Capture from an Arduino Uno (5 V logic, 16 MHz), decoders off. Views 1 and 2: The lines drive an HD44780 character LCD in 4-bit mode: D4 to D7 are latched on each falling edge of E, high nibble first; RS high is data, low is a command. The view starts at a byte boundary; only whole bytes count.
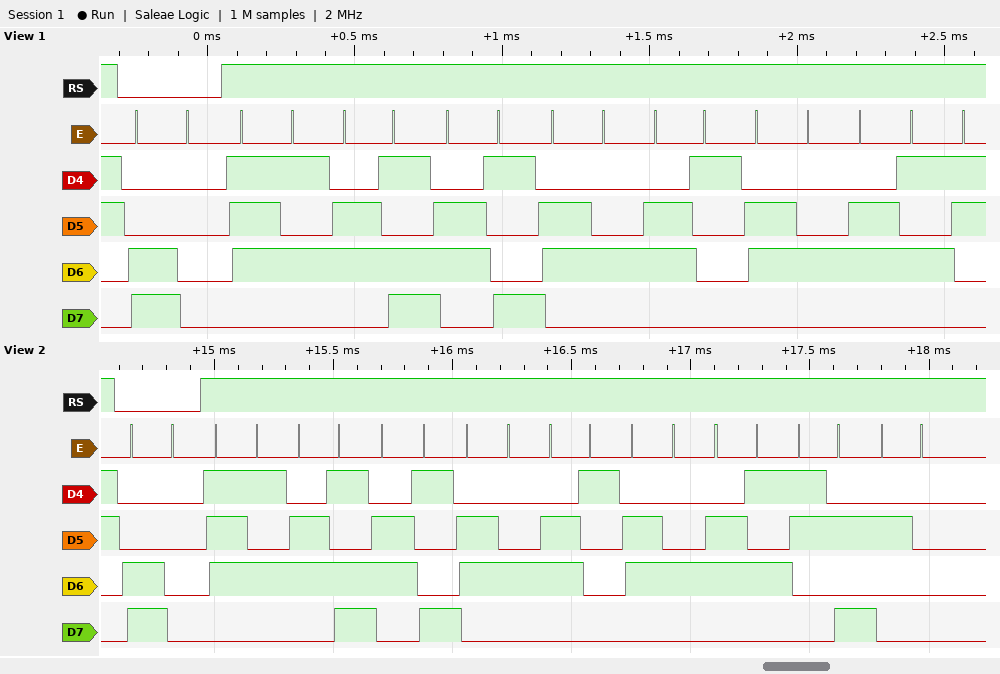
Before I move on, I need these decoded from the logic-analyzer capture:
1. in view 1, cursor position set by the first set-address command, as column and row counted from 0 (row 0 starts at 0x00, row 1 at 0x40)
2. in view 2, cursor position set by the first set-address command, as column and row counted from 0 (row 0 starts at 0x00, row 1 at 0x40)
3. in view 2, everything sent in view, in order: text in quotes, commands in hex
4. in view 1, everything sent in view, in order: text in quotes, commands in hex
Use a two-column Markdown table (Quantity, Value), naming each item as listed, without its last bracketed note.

| Quantity | Value |
|---|---|
| in view 1, cursor position set by the first set-address command, as column and row counted from 0 | column 0, row 1 |
| in view 2, cursor position set by the first set-address command, as column and row counted from 0 | column 0, row 1 |
| in view 2, everything sent in view, in order: text in quotes, commands in hex | 0xC0 "umidade: " |
| in view 1, everything sent in view, in order: text in quotes, commands in hex | 0xC0 "umidade" |
